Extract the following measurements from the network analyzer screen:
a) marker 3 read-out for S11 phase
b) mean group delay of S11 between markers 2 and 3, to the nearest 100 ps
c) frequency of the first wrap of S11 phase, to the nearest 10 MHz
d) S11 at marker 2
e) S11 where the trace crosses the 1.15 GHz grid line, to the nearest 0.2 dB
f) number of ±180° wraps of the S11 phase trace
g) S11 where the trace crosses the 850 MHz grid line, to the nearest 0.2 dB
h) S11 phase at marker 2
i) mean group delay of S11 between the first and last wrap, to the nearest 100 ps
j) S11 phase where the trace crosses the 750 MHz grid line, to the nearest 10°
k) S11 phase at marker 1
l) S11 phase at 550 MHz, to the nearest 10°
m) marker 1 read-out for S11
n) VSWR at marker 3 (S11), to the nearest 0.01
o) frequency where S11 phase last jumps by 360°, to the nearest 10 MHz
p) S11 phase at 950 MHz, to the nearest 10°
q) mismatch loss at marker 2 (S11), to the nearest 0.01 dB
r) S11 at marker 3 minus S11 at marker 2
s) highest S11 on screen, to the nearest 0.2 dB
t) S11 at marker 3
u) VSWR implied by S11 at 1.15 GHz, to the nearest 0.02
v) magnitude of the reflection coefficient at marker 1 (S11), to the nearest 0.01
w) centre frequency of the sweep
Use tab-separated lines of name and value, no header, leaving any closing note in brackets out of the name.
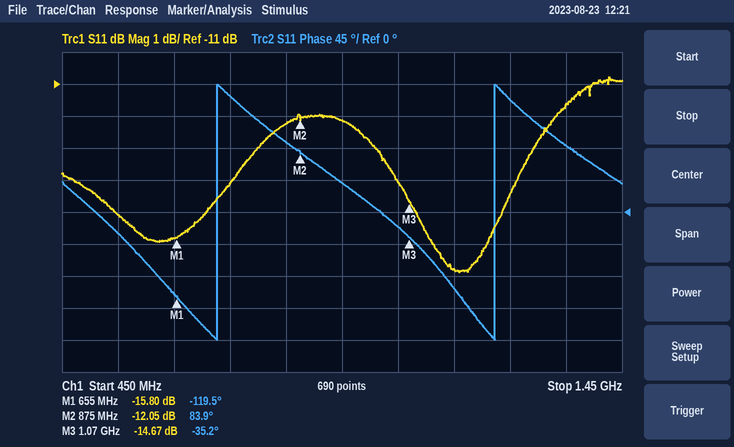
marker 3 read-out for S11 phase	-35.2°
mean group delay of S11 between markers 2 and 3, to the nearest 100 ps	1.7 ns
frequency of the first wrap of S11 phase, to the nearest 10 MHz	730 MHz
S11 at marker 2	-12.05 dB
S11 where the trace crosses the 1.15 GHz grid line, to the nearest 0.2 dB	-16.8 dB
number of ±180° wraps of the S11 phase trace	2
S11 where the trace crosses the 850 MHz grid line, to the nearest 0.2 dB	-12.2 dB
S11 phase at marker 2	83.9°
mean group delay of S11 between the first and last wrap, to the nearest 100 ps	2.0 ns
S11 phase where the trace crosses the 750 MHz grid line, to the nearest 10°	160°
S11 phase at marker 1	-119.5°
S11 phase at 550 MHz, to the nearest 10°	-30°
marker 1 read-out for S11	-15.80 dB
VSWR at marker 3 (S11), to the nearest 0.01	1.45
frequency where S11 phase last jumps by 360°, to the nearest 10 MHz	1.22 GHz
S11 phase at 950 MHz, to the nearest 10°	40°
mismatch loss at marker 2 (S11), to the nearest 0.01 dB	0.28 dB
S11 at marker 3 minus S11 at marker 2	-2.62 dB
highest S11 on screen, to the nearest 0.2 dB	-10.8 dB
S11 at marker 3	-14.67 dB
VSWR implied by S11 at 1.15 GHz, to the nearest 0.02	1.34
magnitude of the reflection coefficient at marker 1 (S11), to the nearest 0.01	0.16
centre frequency of the sweep	950 MHz
